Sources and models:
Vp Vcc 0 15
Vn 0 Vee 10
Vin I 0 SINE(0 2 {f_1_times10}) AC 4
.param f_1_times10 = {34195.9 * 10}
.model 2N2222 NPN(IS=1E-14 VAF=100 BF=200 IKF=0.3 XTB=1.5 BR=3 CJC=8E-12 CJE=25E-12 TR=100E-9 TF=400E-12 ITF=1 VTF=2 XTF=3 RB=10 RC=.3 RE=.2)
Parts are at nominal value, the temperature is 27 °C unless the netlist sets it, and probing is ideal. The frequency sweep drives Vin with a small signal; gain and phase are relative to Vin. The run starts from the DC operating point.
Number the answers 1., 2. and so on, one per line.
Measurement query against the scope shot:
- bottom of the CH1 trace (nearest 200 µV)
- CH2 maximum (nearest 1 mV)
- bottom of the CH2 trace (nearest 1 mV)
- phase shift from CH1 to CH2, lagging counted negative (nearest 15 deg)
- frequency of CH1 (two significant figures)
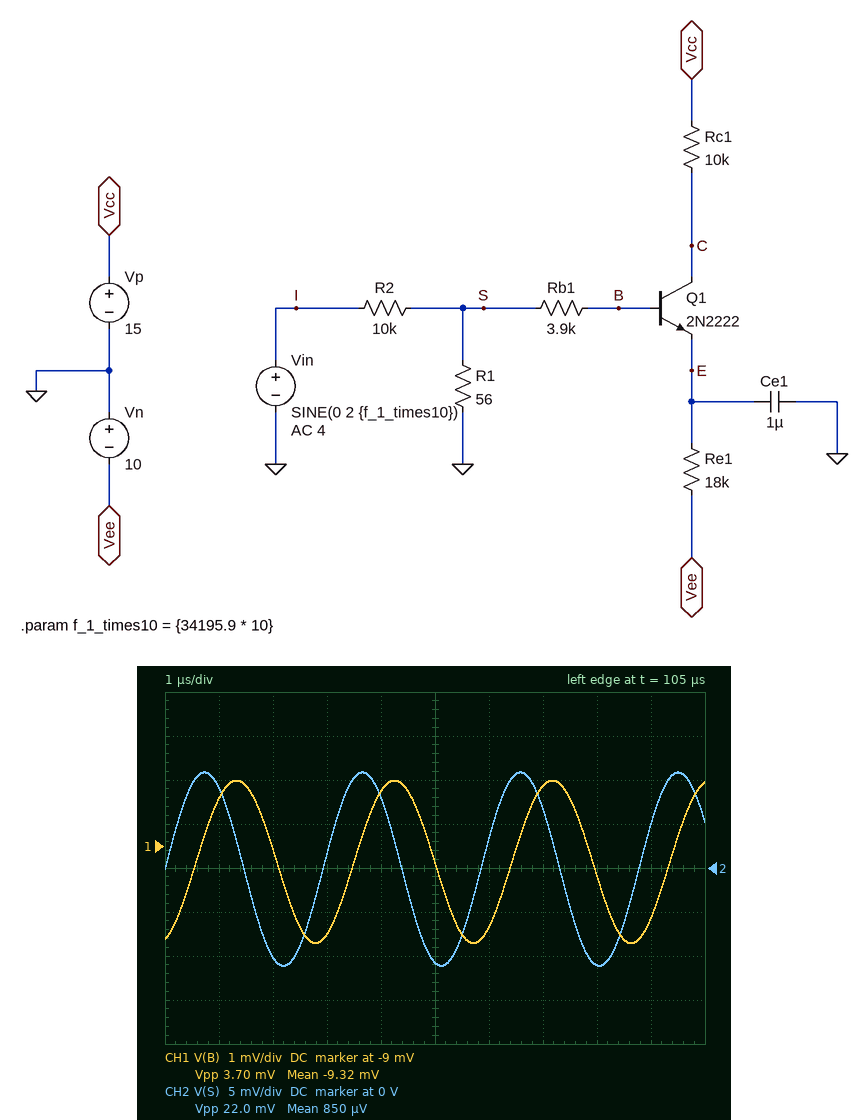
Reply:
1. -11.2 mV
2. 11 mV
3. -11 mV
4. 75 deg
5. 340 kHz
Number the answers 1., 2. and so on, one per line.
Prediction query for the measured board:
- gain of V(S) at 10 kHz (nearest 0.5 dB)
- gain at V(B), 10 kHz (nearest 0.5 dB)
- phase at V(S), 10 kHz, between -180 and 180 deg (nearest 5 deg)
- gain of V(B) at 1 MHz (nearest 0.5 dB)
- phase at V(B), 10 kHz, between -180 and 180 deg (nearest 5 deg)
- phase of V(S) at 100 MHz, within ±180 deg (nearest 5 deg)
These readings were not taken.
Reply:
1. -45.0 dB
2. -47.5 dB
3. 0 deg
4. -69.5 dB
5. -10 deg
6. 0 deg
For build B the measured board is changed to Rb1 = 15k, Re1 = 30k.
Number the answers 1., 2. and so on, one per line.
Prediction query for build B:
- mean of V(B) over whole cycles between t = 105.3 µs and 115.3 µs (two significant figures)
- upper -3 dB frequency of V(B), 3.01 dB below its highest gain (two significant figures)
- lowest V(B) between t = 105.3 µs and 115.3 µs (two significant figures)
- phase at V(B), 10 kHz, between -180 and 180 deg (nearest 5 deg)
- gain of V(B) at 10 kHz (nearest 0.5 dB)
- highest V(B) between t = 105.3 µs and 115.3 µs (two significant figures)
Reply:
1. -21 mV
2. 1.8 kHz
3. -22 mV
4. -15 deg
5. -50.0 dB
6. -20 mV
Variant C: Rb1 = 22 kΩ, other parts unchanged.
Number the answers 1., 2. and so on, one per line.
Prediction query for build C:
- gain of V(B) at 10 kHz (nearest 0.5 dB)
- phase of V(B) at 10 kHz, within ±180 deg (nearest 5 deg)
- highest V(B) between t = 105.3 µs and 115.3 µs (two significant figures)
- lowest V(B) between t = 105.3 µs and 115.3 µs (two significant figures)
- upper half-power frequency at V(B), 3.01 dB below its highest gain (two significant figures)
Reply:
1. -54.5 dB
2. -30 deg
3. -51 mV
4. -52 mV
5. 1.2 kHz
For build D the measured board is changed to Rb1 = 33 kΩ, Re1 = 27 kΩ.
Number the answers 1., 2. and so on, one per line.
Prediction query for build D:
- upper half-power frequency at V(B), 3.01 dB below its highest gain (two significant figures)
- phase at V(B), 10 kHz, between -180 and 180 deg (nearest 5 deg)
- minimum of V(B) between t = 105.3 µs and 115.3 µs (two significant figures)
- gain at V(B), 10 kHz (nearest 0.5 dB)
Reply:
1. 820 Hz
2. -25 deg
3. -51 mV
4. -54.5 dB
